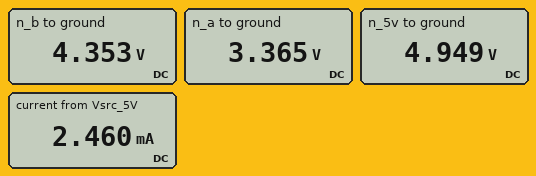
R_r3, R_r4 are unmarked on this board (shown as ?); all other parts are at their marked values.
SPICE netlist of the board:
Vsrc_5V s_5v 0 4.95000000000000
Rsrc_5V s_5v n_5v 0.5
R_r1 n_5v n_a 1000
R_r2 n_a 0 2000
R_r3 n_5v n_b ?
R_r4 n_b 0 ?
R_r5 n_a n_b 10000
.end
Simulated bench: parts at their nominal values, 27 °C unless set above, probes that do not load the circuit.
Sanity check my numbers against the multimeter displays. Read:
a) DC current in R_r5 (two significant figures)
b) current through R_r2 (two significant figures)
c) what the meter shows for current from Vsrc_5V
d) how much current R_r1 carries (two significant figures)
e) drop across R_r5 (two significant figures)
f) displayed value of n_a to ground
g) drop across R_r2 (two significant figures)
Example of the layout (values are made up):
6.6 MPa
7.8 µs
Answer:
99 µA
1.7 mA
2.460 mA
1.6 mA
990 mV
3.365 V
3.4 V
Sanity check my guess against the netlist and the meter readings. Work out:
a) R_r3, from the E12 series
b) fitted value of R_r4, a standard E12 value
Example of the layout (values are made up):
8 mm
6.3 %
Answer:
680 Ω
5.6 kΩ
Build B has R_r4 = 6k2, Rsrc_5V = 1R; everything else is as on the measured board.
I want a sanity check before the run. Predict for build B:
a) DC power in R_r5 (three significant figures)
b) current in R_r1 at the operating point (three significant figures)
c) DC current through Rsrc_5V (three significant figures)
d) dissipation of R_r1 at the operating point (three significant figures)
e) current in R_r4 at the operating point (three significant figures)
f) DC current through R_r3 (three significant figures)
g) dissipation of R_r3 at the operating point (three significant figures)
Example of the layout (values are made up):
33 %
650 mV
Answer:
106 µW
1.58 mA
2.39 mA
2.50 mW
709 µA
812 µA
448 µW
